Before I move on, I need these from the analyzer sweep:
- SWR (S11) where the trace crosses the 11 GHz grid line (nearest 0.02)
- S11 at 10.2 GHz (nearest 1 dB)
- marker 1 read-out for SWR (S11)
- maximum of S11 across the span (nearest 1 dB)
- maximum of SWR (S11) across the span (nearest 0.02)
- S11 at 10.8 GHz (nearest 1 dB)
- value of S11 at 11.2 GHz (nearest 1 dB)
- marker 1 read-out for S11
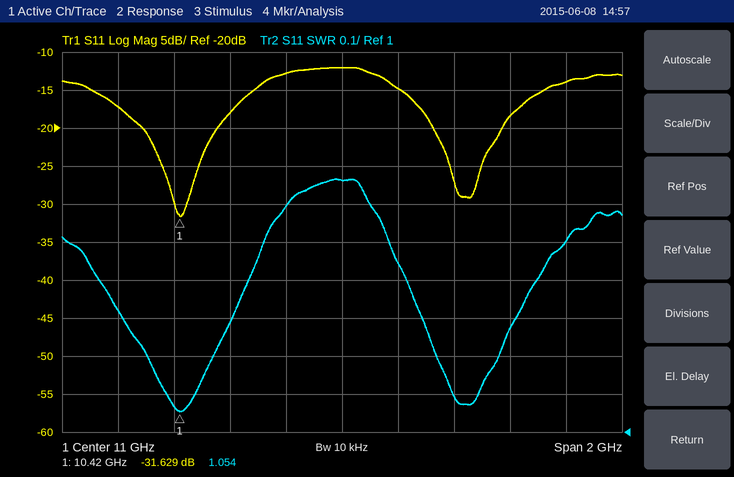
1.66
-17 dB
1.054
-12 dB
1.66
-13 dB
-15 dB
-31.629 dB
